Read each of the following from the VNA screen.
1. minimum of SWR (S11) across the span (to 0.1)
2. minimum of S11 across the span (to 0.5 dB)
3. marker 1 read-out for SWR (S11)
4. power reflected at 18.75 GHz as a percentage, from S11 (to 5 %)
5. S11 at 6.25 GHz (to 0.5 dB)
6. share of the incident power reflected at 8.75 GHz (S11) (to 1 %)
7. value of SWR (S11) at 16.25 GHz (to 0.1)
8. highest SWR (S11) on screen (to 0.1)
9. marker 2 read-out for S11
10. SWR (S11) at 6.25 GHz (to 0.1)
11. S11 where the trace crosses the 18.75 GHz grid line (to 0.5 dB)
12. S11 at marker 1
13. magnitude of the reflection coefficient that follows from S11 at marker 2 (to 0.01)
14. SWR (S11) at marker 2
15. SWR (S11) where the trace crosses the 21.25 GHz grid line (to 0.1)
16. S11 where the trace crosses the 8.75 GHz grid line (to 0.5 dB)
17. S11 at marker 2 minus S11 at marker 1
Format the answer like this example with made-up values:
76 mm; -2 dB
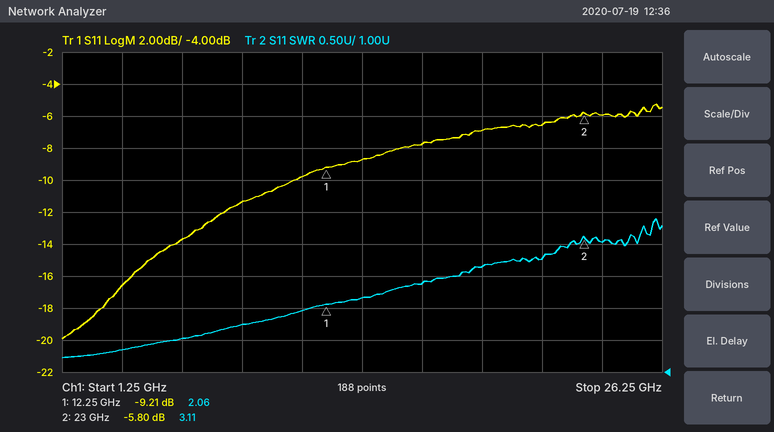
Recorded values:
1.2; -20.0 dB; 2.06; 20 %; -13.5 dB; 7 %; 2.4; 3.4; -5.80 dB; 1.5; -7.0 dB; -9.21 dB; 0.51; 3.11; 2.8; -11.5 dB; 3.41 dB
